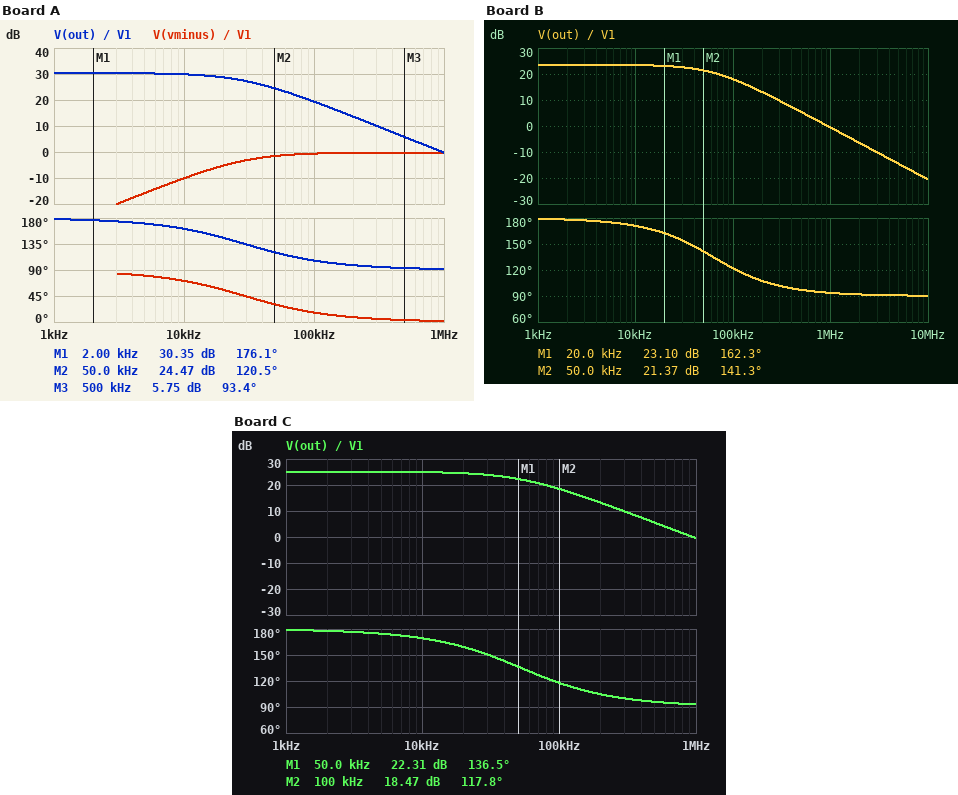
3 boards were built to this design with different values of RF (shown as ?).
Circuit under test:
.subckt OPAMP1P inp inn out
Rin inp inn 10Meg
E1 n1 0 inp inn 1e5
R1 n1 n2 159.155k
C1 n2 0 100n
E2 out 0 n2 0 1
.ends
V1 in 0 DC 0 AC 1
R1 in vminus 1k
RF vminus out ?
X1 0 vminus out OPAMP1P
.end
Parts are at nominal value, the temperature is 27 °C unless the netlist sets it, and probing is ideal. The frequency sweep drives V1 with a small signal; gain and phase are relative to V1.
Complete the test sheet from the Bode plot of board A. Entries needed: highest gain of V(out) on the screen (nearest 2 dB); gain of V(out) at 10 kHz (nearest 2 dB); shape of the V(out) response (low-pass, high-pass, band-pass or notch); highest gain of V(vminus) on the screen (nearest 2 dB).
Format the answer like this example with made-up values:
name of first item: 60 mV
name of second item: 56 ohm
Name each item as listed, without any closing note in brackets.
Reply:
highest gain of V(out) on the screen: 30 dB
gain of V(out) at 10 kHz: 30 dB
shape of the V(out) response: low-pass
highest gain of V(vminus) on the screen: 0 dB
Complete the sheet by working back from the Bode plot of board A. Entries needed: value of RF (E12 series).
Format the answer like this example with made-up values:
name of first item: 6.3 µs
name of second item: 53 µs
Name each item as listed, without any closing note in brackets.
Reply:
value of RF: 33 kΩ
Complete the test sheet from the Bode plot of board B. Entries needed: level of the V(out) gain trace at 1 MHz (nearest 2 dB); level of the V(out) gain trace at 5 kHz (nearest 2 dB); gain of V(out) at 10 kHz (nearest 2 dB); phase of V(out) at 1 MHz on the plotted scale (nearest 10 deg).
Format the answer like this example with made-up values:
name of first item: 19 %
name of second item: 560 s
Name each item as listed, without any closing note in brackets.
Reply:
level of the V(out) gain trace at 1 MHz: 0 dB
level of the V(out) gain trace at 5 kHz: 24 dB
gain of V(out) at 10 kHz: 24 dB
phase of V(out) at 1 MHz on the plotted scale: 90 deg
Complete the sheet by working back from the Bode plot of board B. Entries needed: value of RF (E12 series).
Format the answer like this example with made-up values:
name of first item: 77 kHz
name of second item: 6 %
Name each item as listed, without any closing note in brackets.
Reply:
value of RF: 15 kΩ
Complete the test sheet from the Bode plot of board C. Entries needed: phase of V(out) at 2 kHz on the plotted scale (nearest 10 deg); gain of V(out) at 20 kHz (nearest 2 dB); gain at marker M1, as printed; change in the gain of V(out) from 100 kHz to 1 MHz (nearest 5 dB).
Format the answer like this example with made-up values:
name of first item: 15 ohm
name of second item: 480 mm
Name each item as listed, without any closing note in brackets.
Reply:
phase of V(out) at 2 kHz on the plotted scale: 180 deg
gain of V(out) at 20 kHz: 24 dB
gain at marker M1, as printed: 22.31 dB
change in the gain of V(out) from 100 kHz to 1 MHz: -20 dB
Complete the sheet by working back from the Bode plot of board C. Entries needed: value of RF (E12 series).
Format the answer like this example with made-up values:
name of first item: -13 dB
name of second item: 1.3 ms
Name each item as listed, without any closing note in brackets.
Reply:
value of RF: 18 kΩ
